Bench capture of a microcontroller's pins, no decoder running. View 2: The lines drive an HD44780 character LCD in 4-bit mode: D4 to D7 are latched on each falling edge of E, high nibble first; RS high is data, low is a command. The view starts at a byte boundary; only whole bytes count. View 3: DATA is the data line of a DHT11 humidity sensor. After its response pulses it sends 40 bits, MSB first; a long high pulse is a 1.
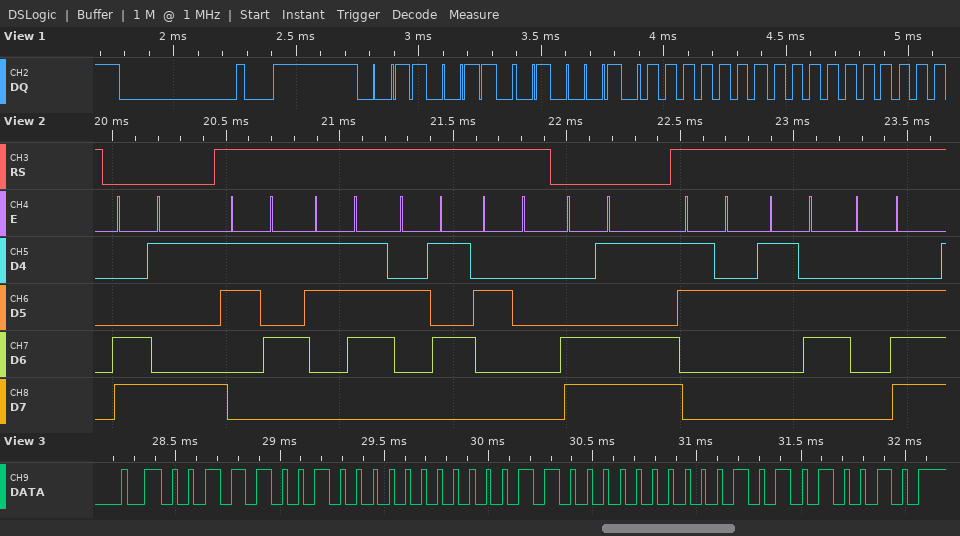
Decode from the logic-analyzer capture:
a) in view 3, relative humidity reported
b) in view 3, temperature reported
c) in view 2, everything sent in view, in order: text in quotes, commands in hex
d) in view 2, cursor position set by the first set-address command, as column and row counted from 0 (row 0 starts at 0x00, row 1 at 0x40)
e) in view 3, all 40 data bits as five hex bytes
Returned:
57 %
24.1 °C
0xC9 "57% " 0xCD "26."
column 9, row 1
39 00 18 01 52
